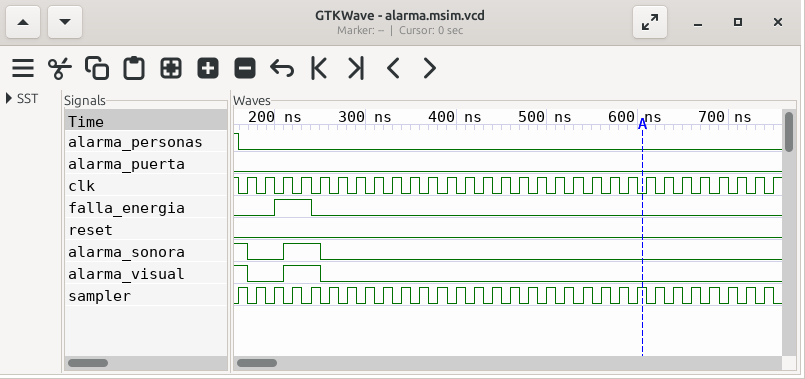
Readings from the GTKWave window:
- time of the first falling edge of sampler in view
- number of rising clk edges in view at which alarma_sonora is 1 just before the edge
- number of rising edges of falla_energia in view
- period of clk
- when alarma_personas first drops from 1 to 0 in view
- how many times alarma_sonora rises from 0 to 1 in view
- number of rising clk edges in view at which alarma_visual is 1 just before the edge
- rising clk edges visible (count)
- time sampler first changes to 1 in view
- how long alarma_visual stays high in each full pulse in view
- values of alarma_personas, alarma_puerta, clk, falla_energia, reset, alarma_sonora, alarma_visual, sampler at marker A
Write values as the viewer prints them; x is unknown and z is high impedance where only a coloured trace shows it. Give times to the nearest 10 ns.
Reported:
170 ns
3
1
20 ns
160 ns
1
3
30
160 ns
40 ns
alarma_personas=0, alarma_puerta=0, clk=0, falla_energia=0, reset=0, alarma_sonora=0, alarma_visual=0, sampler=1
